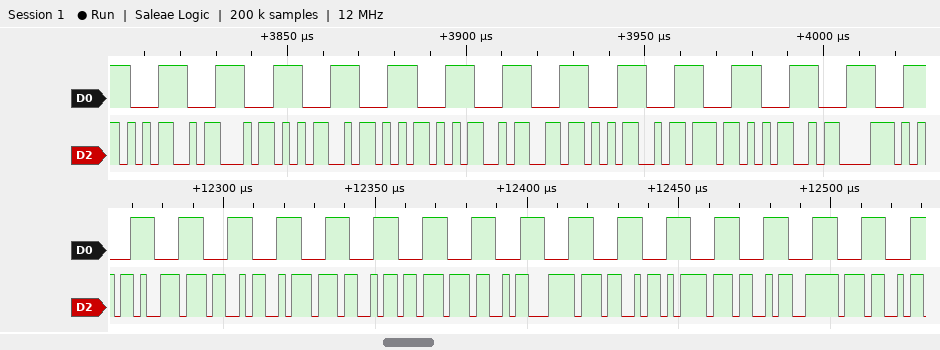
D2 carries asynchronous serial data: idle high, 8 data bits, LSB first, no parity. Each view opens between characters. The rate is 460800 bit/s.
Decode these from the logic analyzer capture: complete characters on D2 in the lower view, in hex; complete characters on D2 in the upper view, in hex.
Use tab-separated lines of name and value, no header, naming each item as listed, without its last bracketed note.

complete characters on D2 in the lower view, in hex	CB, 37, D3, 37, DB, 37, E3, 37, EB, 37, F3, 37
complete characters on D2 in the upper view, in hex	35, A3, 35, AB, 35, B3, 35, BB, 35, C3
